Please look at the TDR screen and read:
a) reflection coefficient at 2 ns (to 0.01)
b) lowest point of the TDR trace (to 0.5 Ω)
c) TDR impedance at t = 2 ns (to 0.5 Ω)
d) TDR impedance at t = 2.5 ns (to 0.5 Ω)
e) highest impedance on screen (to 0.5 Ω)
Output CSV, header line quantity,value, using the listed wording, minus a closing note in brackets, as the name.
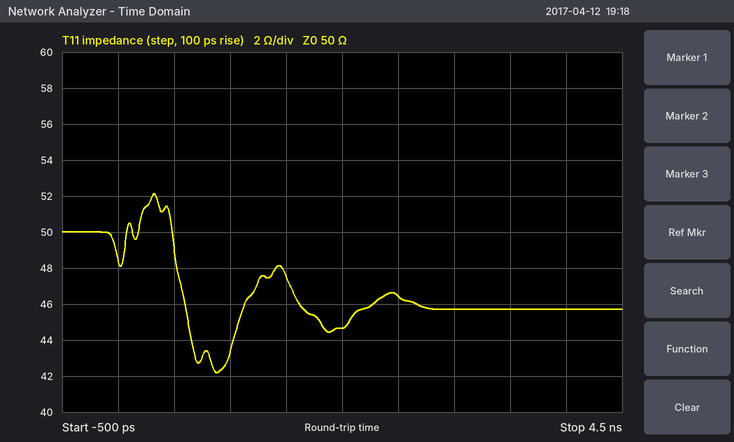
quantity,value
reflection coefficient at 2 ns,-0.06
lowest point of the TDR trace,42.0 Ω
TDR impedance at t = 2 ns,44.5 Ω
TDR impedance at t = 2.5 ns,46.5 Ω
highest impedance on screen,52.0 Ω
